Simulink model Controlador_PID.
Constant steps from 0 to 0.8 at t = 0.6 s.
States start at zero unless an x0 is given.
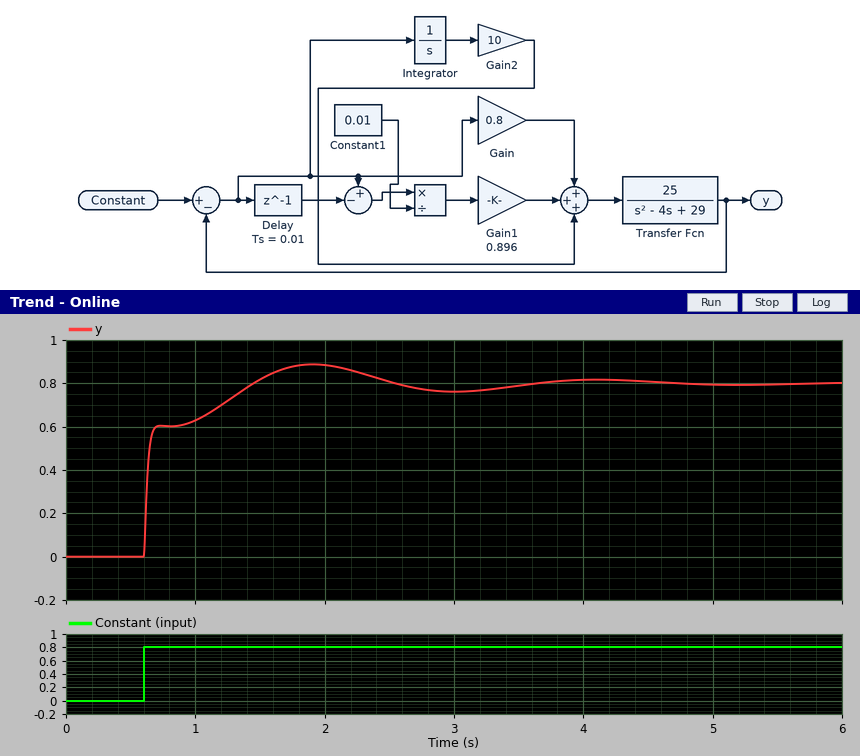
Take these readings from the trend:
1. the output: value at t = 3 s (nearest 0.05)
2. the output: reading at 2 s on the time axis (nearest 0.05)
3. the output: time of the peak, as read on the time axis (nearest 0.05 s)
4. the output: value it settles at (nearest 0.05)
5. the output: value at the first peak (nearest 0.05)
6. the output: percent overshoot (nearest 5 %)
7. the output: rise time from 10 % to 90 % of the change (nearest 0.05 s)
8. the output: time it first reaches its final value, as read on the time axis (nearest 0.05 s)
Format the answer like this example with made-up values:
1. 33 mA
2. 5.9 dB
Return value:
1. 0.75
2. 0.90
3. 1.90 s
4. 0.80
5. 0.90
6. 10 %
7. 0.65 s
8. 1.45 s
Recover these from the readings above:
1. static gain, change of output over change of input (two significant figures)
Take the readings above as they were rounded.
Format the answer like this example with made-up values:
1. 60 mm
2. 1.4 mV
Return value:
1. 1.0
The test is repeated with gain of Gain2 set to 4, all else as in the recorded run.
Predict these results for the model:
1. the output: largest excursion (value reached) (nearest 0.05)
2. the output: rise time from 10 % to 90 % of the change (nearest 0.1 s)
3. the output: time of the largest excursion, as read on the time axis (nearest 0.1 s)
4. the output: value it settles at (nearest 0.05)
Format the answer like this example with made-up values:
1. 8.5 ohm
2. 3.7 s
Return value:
1. 0.85
2. 1.3 s
3. 2.9 s
4. 0.80
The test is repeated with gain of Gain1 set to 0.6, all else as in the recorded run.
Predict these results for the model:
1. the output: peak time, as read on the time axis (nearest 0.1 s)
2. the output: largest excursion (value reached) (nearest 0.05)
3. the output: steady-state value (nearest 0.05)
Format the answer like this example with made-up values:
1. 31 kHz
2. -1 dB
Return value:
1. 1.7 s
2. 0.85
3. 0.80
